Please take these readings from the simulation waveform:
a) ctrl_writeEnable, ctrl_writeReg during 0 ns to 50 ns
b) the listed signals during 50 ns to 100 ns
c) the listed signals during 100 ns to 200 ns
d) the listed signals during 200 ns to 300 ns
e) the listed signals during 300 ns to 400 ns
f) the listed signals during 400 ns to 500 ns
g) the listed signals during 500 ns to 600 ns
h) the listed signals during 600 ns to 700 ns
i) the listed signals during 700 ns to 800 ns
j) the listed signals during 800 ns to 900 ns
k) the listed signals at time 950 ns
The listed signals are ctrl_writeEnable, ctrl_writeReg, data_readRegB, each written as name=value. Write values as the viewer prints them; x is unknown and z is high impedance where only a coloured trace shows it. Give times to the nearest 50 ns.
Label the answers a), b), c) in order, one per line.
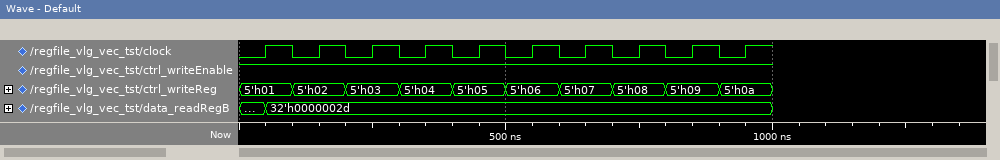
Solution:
a) ctrl_writeEnable=1, ctrl_writeReg=5'h01
b) ctrl_writeEnable=1, ctrl_writeReg=5'h01, data_readRegB=32'h0000002d
c) ctrl_writeEnable=1, ctrl_writeReg=5'h02, data_readRegB=32'h0000002d
d) ctrl_writeEnable=1, ctrl_writeReg=5'h03, data_readRegB=32'h0000002d
e) ctrl_writeEnable=1, ctrl_writeReg=5'h04, data_readRegB=32'h0000002d
f) ctrl_writeEnable=1, ctrl_writeReg=5'h05, data_readRegB=32'h0000002d
g) ctrl_writeEnable=1, ctrl_writeReg=5'h06, data_readRegB=32'h0000002d
h) ctrl_writeEnable=1, ctrl_writeReg=5'h07, data_readRegB=32'h0000002d
i) ctrl_writeEnable=1, ctrl_writeReg=5'h08, data_readRegB=32'h0000002d
j) ctrl_writeEnable=1, ctrl_writeReg=5'h09, data_readRegB=32'h0000002d
k) ctrl_writeEnable=1, ctrl_writeReg=5'h0a, data_readRegB=32'h0000002d
